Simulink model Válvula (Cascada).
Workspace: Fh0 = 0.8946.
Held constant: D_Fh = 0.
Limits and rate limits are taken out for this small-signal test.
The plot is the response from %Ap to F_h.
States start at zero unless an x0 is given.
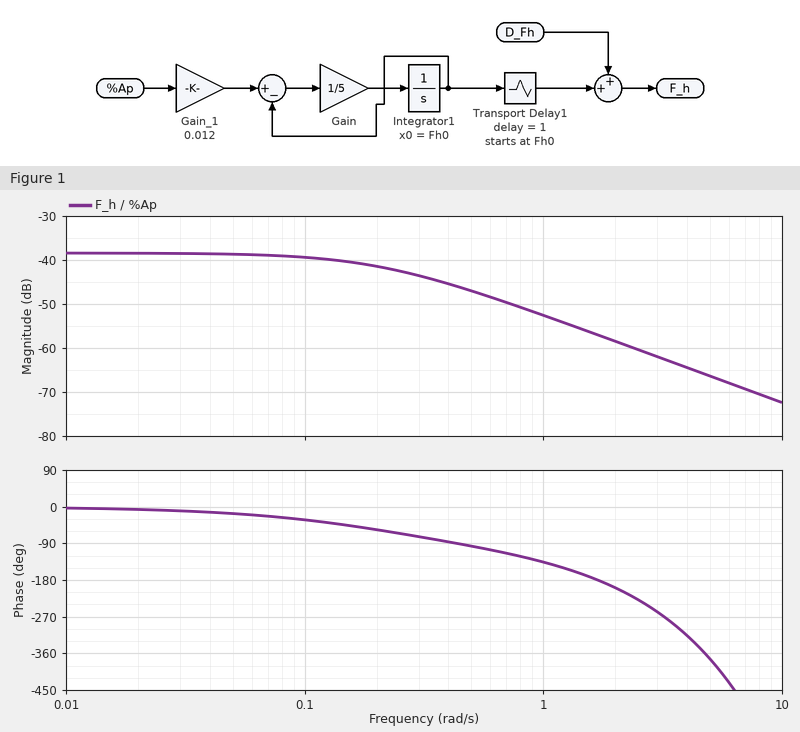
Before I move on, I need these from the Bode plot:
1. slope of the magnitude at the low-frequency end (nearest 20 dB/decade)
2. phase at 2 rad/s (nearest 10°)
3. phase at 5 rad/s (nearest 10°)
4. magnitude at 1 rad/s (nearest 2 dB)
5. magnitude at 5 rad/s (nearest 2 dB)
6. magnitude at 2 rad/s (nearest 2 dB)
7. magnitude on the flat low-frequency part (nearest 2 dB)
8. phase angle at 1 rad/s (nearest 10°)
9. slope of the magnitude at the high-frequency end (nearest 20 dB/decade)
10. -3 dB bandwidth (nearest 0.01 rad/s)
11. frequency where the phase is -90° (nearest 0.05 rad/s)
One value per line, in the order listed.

0 dB/decade
-200°
-370°
-52 dB
-66 dB
-58 dB
-38 dB
-140°
-20 dB/decade
0.20 rad/s
0.45 rad/s
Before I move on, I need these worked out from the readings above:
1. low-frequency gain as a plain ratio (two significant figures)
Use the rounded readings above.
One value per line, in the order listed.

0.013
